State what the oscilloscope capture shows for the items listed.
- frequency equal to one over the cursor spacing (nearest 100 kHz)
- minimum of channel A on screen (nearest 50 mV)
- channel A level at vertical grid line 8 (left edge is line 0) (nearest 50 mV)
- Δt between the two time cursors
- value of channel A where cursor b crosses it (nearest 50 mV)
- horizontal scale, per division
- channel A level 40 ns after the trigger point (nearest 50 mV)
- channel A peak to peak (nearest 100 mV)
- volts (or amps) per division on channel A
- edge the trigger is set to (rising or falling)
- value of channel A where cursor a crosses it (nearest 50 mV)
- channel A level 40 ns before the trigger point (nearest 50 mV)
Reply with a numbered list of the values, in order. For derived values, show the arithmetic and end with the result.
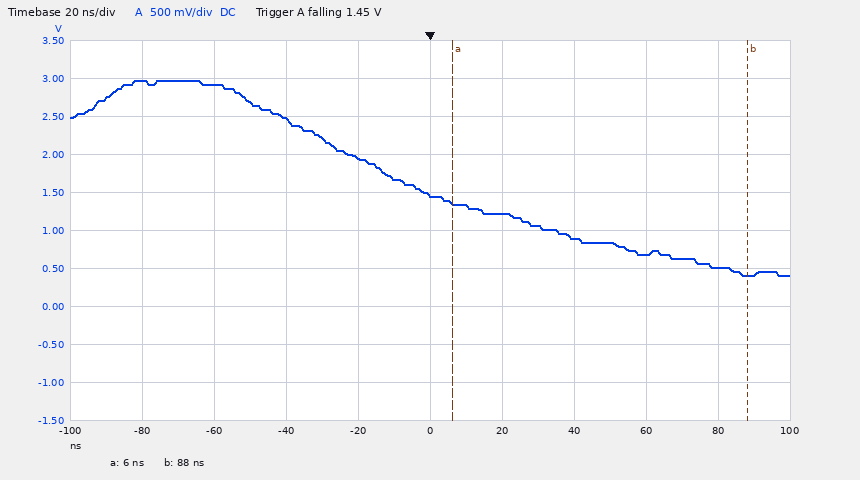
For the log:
1. 1 / 82 ns ≈ 12.2 MHz
2. 400 mV
3. 700 mV
4. 88 ns − (6 ns) = 82 ns
5. 400 mV
6. 20 ns
7. 900 mV
8. 2.60 V
9. 500 mV
10. falling
11. 1.35 V
12. 2.45 V
